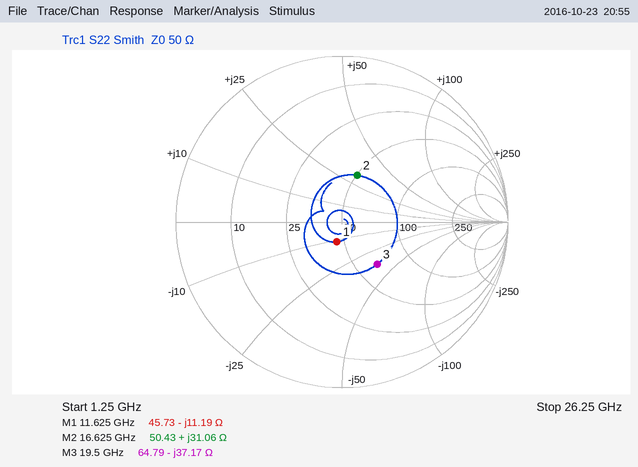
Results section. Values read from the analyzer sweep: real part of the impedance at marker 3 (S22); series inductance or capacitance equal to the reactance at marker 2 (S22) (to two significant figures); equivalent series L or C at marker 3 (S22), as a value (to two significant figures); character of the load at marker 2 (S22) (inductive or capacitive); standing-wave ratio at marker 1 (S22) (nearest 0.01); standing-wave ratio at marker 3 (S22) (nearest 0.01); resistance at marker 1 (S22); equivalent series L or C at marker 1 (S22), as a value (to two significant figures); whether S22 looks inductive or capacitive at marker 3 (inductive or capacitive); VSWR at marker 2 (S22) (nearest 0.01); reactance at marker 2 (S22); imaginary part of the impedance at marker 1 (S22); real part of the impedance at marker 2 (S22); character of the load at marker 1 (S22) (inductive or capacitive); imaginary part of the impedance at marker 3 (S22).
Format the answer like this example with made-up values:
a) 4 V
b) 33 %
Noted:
a) 64.79 Ω
b) 300 pH
c) 220 fF
d) inductive
e) 1.28
f) 1.99
g) 45.73 Ω
h) 1.2 pF
i) capacitive
j) 1.84
k) +31.06 Ω
l) -11.19 Ω
m) 50.43 Ω
n) capacitive
o) -37.17 Ω
